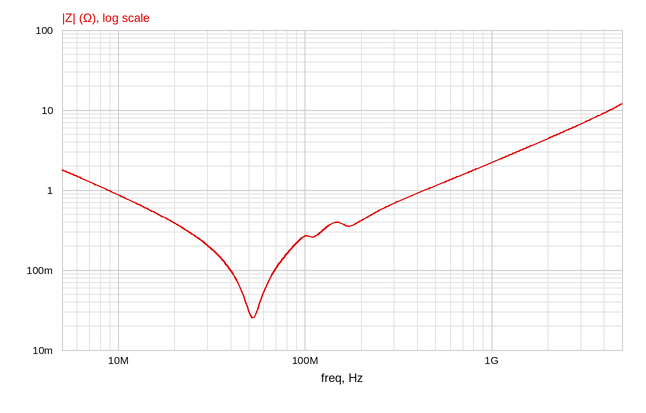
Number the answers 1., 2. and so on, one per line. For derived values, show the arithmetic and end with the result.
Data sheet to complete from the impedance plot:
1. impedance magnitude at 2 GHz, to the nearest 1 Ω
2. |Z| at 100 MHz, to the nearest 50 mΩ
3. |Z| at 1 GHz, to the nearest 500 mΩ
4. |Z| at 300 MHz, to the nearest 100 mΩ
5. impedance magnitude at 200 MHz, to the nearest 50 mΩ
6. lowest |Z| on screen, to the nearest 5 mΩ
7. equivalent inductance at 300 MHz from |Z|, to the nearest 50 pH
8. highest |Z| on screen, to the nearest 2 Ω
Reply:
1. 4 Ω
2. 250 mΩ
3. 2.0 Ω
4. 700 mΩ
5. 400 mΩ
6. 25 mΩ
7. L = 700 mΩ/(2π × 300 MHz) ≈ 371 pH, so 350 pH to the nearest 50 pH
8. 12 Ω
